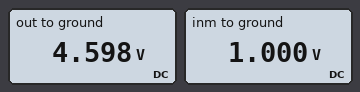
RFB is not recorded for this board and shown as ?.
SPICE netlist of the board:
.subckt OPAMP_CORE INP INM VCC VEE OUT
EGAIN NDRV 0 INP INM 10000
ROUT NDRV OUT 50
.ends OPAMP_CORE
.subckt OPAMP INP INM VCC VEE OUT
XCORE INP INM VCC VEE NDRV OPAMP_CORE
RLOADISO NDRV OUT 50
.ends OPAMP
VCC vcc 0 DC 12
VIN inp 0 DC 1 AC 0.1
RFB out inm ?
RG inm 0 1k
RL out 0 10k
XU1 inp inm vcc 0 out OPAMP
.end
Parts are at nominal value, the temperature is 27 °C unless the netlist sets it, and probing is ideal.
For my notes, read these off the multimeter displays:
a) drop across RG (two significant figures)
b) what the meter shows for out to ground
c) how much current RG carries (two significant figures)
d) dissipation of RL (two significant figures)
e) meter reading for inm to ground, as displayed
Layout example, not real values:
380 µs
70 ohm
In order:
1.0 V
4.598 V
1.0 mA
2.1 mW
1.000 V
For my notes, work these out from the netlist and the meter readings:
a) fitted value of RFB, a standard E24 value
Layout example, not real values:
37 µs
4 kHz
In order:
3.6 kΩ
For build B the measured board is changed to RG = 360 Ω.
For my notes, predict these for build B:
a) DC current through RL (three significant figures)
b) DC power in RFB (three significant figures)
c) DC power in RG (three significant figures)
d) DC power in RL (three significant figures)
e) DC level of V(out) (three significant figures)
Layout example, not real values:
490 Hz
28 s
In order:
1.10 mA
27.7 mW
2.77 mW
12.1 mW
11.0 V
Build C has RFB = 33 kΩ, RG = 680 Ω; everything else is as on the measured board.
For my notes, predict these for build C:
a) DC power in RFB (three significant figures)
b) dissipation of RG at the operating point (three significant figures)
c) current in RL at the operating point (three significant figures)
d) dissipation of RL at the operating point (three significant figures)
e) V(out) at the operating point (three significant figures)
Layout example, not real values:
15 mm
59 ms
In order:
70.7 mW
1.46 mW
4.93 mA
243 mW
49.3 V
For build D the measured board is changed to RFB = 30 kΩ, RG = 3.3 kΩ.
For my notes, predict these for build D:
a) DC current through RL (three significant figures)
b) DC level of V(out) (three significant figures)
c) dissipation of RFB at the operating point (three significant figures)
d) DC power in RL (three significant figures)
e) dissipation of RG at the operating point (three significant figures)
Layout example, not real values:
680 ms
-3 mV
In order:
1.01 mA
10.1 V
2.75 mW
10.2 mW
302 µW
